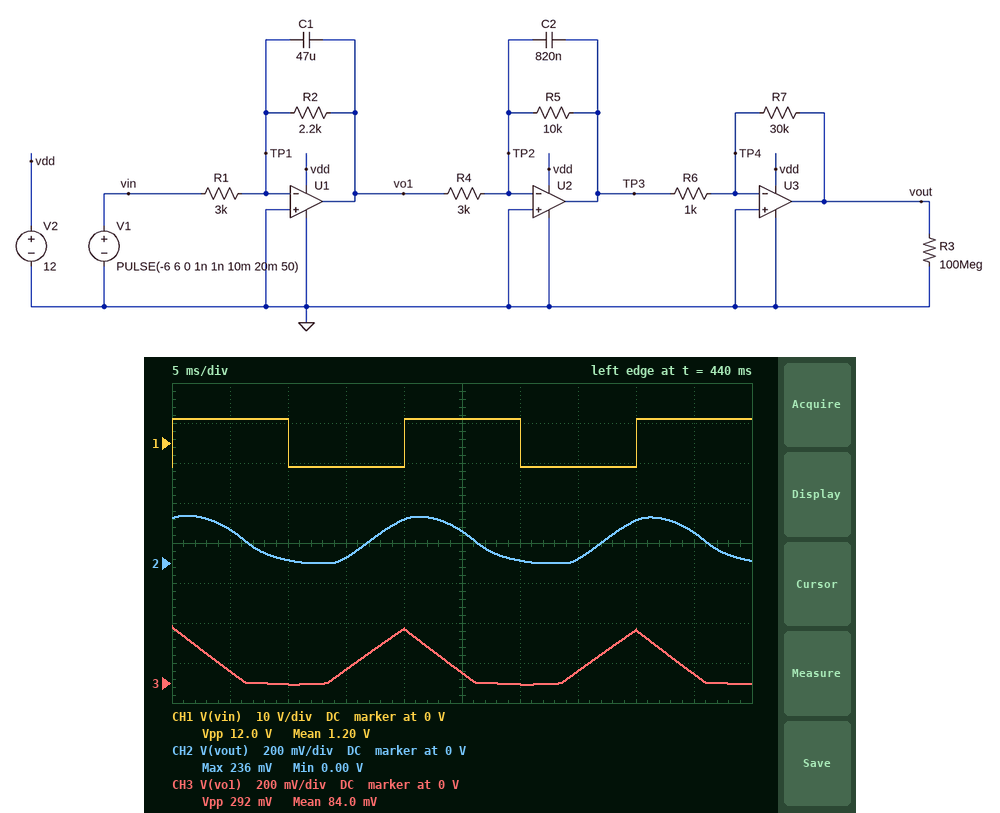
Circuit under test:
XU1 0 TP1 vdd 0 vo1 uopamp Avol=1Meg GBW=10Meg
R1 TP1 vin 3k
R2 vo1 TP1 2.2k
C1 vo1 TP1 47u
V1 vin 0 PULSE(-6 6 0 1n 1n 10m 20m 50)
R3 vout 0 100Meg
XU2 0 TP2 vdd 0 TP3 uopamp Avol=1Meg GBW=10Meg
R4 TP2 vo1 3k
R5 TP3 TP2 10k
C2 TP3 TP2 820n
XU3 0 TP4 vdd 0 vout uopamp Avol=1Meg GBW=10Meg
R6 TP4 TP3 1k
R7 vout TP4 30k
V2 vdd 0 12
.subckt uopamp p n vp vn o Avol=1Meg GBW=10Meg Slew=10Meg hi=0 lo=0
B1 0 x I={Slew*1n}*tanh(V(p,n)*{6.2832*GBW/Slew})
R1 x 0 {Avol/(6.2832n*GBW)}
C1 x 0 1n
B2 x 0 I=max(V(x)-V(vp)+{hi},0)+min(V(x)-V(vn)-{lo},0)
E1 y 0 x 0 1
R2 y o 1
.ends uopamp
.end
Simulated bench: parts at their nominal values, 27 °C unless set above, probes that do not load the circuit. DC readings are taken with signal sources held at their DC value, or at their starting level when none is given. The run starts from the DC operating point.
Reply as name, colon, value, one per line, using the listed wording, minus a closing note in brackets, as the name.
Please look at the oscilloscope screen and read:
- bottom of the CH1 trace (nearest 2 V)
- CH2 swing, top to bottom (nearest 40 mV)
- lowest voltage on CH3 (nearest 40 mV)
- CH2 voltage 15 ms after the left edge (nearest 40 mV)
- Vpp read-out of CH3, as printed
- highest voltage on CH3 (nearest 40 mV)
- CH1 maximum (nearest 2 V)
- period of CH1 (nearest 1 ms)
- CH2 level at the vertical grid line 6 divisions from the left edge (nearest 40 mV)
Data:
bottom of the CH1 trace: -6 V
CH2 swing, top to bottom: 240 mV
lowest voltage on CH3: 0 V
CH2 voltage 15 ms after the left edge: 40 mV
Vpp read-out of CH3, as printed: 292 mV
highest voltage on CH3: 280 mV
CH1 maximum: 6 V
period of CH1: 20 ms
CH2 level at the vertical grid line 6 divisions from the left edge: 0 V
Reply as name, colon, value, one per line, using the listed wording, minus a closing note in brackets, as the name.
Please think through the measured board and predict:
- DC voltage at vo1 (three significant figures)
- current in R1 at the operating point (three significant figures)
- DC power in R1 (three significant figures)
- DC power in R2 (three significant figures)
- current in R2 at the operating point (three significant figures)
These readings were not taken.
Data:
DC voltage at vo1: 4.40 V
current in R1 at the operating point: 2.00 mA
DC power in R1: 12.0 mW
DC power in R2: 8.80 mW
current in R2 at the operating point: 2.00 mA
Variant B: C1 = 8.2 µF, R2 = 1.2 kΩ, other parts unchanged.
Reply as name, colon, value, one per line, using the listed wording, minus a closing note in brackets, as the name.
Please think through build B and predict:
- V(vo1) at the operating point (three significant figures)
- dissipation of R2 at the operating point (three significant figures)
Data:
V(vo1) at the operating point: 2.40 V
dissipation of R2 at the operating point: 4.80 mW
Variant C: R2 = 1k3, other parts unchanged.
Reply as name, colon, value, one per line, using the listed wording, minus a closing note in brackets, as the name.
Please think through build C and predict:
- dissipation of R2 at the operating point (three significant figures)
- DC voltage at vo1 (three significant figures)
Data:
dissipation of R2 at the operating point: 5.20 mW
DC voltage at vo1: 2.60 V
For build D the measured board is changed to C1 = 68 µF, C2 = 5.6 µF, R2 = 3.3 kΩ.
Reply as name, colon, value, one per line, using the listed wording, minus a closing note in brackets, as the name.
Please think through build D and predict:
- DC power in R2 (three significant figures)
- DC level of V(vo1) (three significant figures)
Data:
DC power in R2: 13.2 mW
DC level of V(vo1): 6.60 V
